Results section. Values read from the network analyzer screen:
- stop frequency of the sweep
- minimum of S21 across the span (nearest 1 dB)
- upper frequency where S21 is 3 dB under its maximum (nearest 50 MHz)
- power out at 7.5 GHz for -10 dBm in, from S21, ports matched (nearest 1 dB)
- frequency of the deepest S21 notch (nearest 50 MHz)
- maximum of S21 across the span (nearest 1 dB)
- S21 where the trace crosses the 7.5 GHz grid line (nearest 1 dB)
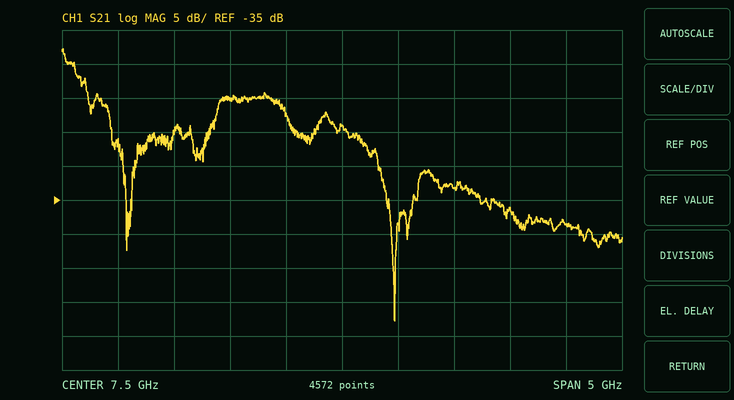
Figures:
10 GHz
-53 dB
5.10 GHz
-34 dBm
7.95 GHz
-13 dB
-24 dB
